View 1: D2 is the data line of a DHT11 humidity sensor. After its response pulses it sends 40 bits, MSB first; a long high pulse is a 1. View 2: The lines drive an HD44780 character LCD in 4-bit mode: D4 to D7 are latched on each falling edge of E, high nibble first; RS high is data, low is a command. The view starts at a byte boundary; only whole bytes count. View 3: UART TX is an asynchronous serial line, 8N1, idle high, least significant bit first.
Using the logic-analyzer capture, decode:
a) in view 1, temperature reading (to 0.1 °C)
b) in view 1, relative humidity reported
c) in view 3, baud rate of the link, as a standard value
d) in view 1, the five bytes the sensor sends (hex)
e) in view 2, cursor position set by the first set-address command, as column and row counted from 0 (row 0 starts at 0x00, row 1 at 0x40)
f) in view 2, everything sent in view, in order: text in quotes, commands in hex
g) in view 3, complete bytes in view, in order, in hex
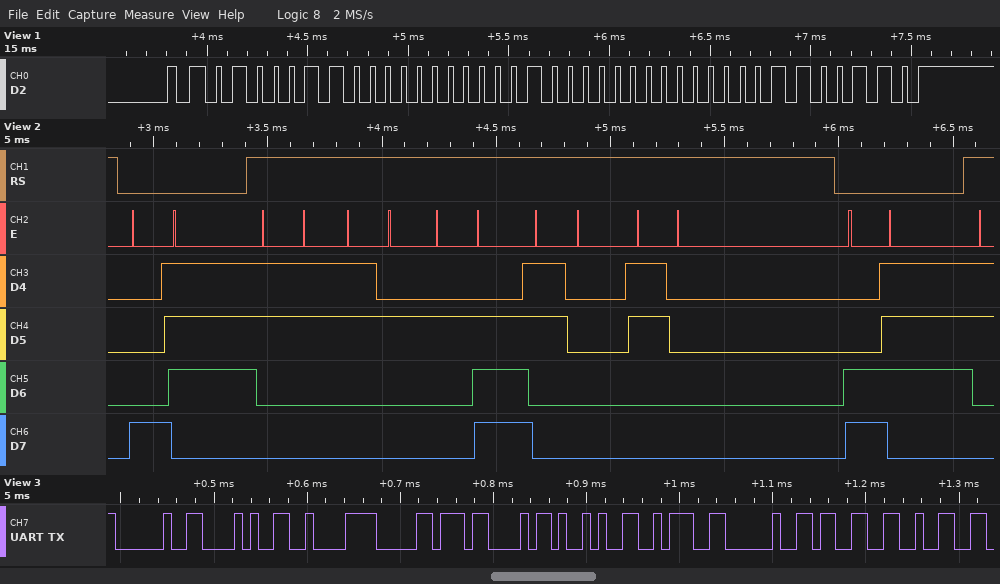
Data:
32.0 °C
70 %
115200 baud
46 00 20 00 66
column 7, row 0
0x87 "32.00" 0xC7
20 28 C2 B0 43 29 3A 20 33 32
